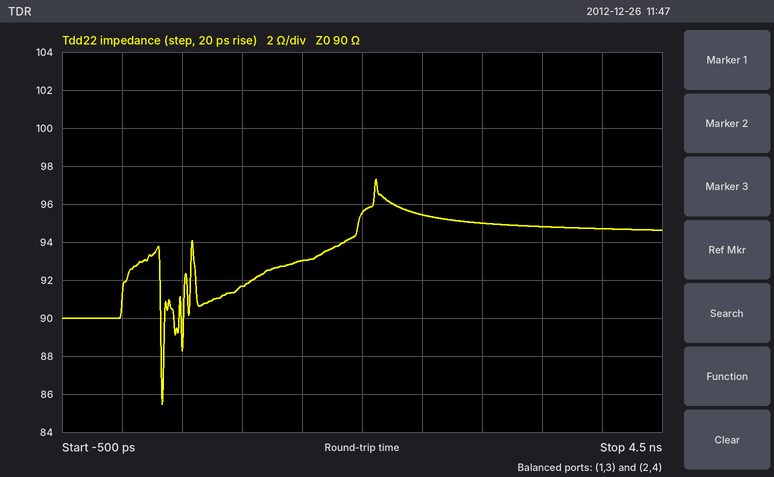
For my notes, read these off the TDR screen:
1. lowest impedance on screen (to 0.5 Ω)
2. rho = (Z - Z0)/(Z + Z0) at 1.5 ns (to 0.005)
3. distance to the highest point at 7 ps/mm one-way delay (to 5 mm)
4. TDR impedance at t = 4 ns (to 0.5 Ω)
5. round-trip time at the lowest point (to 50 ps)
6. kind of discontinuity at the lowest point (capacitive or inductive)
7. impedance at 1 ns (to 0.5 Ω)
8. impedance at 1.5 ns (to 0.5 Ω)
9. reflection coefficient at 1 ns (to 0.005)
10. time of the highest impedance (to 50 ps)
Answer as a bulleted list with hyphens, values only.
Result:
- 85.5 Ω
- +0.015
- 150 mm
- 94.5 Ω
- 350 ps
- capacitive
- 91.5 Ω
- 93.0 Ω
- +0.010
- 2.10 ns
